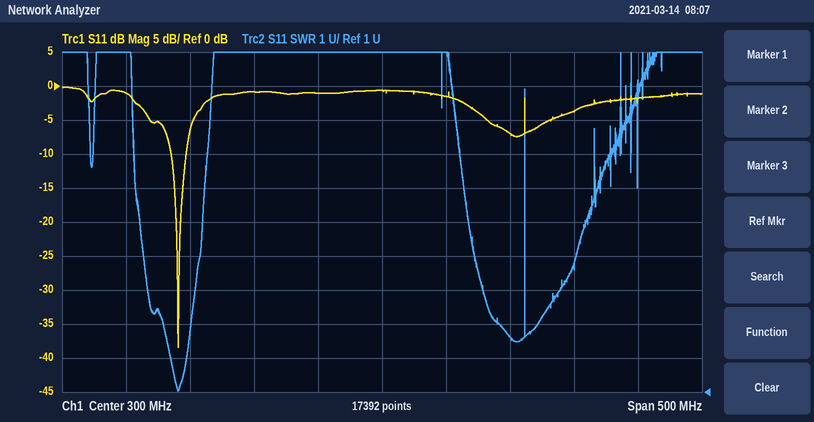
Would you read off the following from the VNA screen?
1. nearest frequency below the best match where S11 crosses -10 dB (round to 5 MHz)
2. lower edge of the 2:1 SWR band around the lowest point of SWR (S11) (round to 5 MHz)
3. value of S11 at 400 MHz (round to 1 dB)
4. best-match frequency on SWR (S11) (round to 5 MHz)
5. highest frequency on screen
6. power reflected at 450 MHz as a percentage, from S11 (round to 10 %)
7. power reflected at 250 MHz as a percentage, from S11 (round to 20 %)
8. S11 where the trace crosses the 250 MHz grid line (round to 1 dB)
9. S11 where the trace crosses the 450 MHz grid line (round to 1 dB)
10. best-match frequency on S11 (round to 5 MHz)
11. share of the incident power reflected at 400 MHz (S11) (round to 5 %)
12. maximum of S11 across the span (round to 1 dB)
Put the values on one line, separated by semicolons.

135 MHz; 135 MHz; -7 dB; 140 MHz; 550 MHz; 40 %; 80 %; -1 dB; -4 dB; 140 MHz; 20 %; 0 dB
